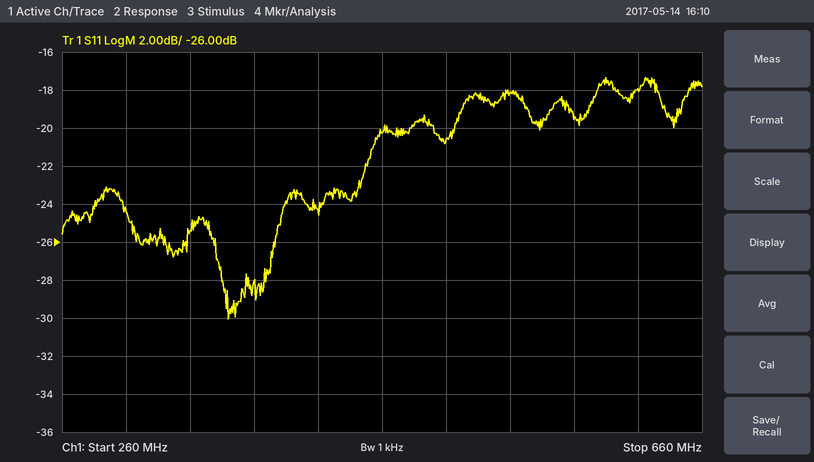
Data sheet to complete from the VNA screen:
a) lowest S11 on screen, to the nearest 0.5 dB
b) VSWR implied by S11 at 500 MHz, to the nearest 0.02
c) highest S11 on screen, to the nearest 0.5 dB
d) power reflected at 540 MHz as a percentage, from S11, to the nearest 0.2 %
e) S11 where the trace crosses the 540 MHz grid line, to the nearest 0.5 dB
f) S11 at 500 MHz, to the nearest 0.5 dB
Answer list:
-30.0 dB
1.20
-17.5 dB
1.6 %
-18.0 dB
-20.5 dB
